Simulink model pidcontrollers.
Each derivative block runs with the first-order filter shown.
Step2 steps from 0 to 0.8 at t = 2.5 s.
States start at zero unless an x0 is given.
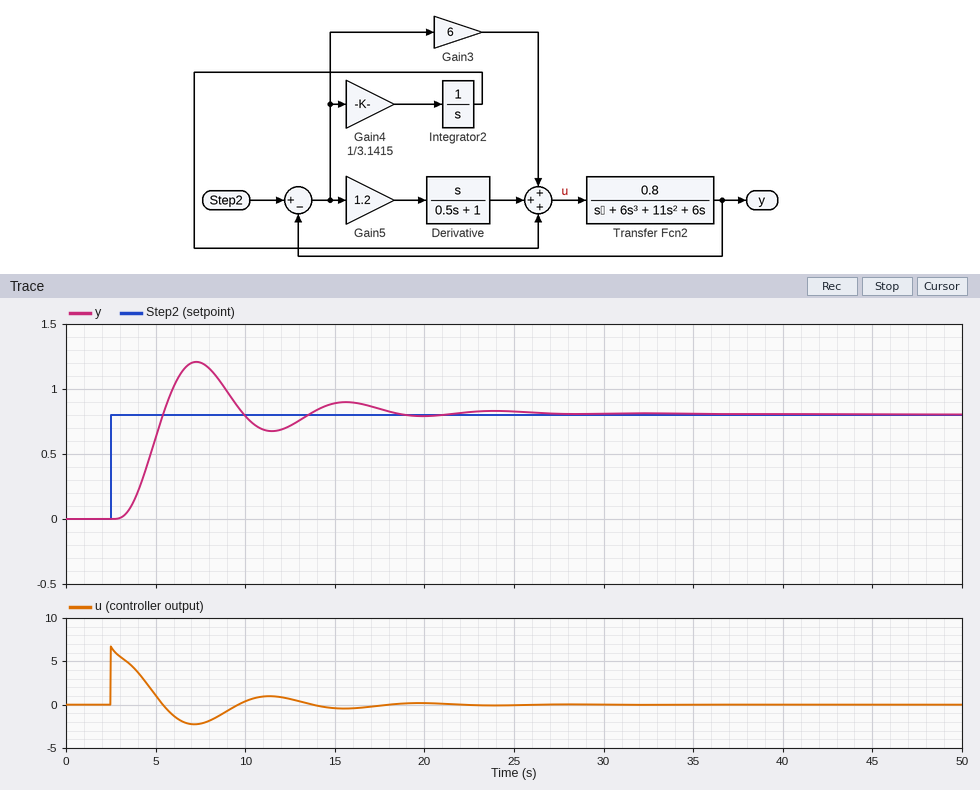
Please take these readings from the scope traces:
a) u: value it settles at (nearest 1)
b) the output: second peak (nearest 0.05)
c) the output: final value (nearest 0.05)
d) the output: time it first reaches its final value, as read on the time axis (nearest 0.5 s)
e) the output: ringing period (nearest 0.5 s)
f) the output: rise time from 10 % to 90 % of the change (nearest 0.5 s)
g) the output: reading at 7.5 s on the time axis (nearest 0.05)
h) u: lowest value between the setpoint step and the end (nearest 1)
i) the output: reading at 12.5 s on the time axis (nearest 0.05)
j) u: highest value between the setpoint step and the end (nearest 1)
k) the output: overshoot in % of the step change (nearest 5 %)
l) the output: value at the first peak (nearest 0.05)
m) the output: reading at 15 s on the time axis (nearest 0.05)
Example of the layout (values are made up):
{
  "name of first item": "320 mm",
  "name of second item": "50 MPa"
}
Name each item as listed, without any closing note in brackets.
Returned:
{
  "u: value it settles at": "0",
  "the output: second peak": "0.90",
  "the output: final value": "0.80",
  "the output: time it first reaches its final value, as read on the time axis": "5.5 s",
  "the output: ringing period": "8.5 s",
  "the output: rise time from 10 % to 90 % of the change": "1.5 s",
  "the output: reading at 7.5 s on the time axis": "1.20",
  "u: lowest value between the setpoint step and the end": "-2",
  "the output: reading at 12.5 s on the time axis": "0.70",
  "u: highest value between the setpoint step and the end": "7",
  "the output: overshoot in % of the step change": "50 %",
  "the output: value at the first peak": "1.20",
  "the output: reading at 15 s on the time axis": "0.90"
}
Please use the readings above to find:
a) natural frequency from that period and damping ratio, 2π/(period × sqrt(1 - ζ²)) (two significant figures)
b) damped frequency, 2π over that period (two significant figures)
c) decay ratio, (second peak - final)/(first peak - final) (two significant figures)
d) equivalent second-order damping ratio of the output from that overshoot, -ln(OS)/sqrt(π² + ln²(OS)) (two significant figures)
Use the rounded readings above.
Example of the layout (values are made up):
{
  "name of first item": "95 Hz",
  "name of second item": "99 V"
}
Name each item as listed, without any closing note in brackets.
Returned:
{
  "natural frequency from that period and damping ratio, 2π/(period × sqrt(1 - ζ²))": "0.76 rad/s",
  "damped frequency, 2π over that period": "0.74 rad/s",
  "decay ratio, (second peak - final)/(first peak - final)": "0.25",
  "equivalent second-order damping ratio of the output from that overshoot, -ln(OS)/sqrt(π² + ln²(OS))": "0.22"
}
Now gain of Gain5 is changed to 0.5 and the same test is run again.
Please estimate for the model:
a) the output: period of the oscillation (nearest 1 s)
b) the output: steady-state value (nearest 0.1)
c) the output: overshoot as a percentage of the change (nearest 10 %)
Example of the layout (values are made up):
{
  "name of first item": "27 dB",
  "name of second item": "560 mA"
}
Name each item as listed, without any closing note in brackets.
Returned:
{
  "the output: period of the oscillation": "9 s",
  "the output: steady-state value": "0.8",
  "the output: overshoot as a percentage of the change": "60 %"
}
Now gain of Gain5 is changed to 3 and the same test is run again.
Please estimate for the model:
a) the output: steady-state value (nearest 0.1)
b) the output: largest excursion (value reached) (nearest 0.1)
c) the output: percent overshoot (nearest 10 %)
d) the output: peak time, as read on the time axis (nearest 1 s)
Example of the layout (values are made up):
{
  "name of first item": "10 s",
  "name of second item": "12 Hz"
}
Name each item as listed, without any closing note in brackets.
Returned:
{
  "the output: steady-state value": "0.8",
  "the output: largest excursion (value reached)": "1.1",
  "the output: percent overshoot": "40 %",
  "the output: peak time, as read on the time axis": "7 s"
}
